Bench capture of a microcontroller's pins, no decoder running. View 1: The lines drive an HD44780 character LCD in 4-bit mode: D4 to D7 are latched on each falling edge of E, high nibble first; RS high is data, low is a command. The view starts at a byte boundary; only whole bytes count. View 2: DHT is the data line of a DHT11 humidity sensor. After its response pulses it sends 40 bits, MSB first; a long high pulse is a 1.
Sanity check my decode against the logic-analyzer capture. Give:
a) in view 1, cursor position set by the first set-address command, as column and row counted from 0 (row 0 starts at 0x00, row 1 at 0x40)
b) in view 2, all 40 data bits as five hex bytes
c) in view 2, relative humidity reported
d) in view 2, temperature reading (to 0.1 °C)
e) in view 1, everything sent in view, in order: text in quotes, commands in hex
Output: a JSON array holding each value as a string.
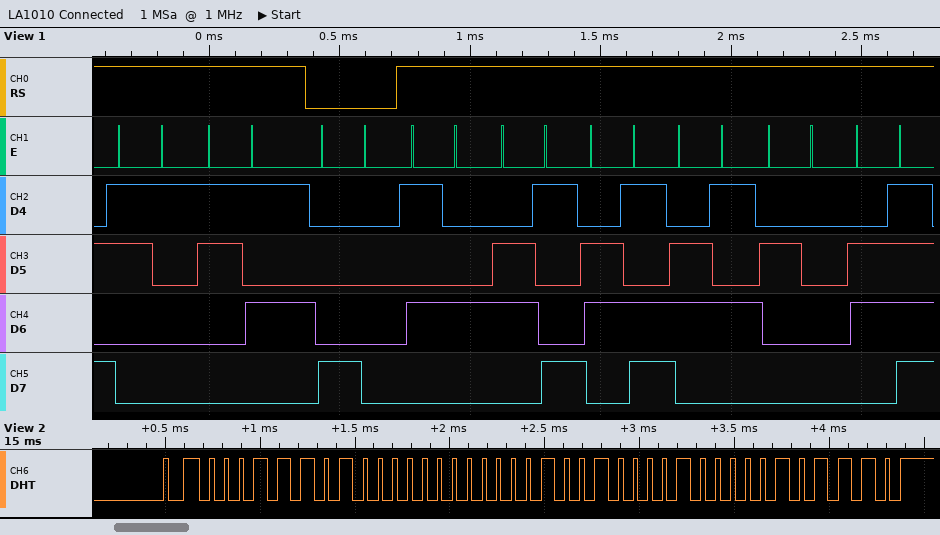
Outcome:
["column 0, row 0", "1D 00 09 08 2E", "29 %", "9.8 °C", "\"15\" 0x80 \"Time o\""]
